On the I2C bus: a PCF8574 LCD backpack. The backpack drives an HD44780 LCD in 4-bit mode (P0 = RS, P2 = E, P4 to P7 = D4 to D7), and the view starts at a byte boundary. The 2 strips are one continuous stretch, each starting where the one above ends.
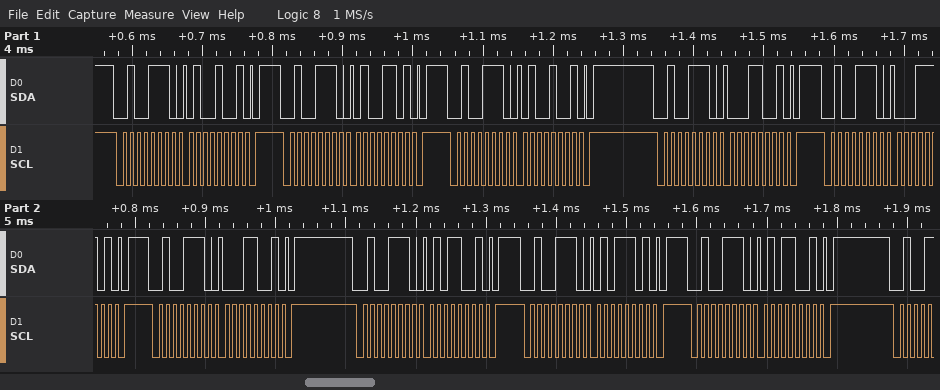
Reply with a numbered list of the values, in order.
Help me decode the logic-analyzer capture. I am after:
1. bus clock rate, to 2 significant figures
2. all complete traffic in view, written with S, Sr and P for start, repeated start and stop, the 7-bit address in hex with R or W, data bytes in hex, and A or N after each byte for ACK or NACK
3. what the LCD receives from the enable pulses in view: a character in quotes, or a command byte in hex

1. 100 kHz
2. S 27W A 49 A P S 27W A 4D A P S 27W A 49 A P S 27W A 19 A P S 27W A 1D A P S 27W A 19 A P S 27W A 59 A P S 27W A 5D A P S 27W A 59 A P
3. 'A'
